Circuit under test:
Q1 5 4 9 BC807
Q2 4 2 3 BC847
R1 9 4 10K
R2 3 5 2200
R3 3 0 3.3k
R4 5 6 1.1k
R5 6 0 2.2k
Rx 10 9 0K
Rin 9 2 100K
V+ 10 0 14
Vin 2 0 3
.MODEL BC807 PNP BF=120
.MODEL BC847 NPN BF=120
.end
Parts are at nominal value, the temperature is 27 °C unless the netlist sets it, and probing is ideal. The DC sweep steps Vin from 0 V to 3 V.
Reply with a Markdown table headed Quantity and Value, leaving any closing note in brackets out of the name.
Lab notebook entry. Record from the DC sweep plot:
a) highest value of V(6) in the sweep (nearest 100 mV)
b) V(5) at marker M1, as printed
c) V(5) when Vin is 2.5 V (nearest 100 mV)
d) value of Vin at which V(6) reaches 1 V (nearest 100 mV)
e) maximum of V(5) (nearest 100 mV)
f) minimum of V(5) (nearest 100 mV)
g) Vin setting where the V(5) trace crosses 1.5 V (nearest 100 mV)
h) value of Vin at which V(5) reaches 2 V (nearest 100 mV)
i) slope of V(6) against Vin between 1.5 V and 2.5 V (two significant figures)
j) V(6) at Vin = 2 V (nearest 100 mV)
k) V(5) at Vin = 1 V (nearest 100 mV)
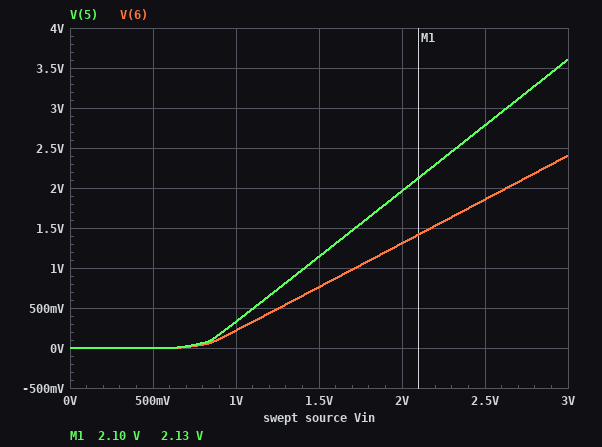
| Quantity | Value |
|---|---|
| highest value of V(6) in the sweep | 2.4 V |
| V(5) at marker M1, as printed | 2.13 V |
| V(5) when Vin is 2.5 V | 2.8 V |
| value of Vin at which V(6) reaches 1 V | 1.7 V |
| maximum of V(5) | 3.6 V |
| minimum of V(5) | 0 V |
| Vin setting where the V(5) trace crosses 1.5 V | 1.7 V |
| value of Vin at which V(5) reaches 2 V | 2.0 V |
| slope of V(6) against Vin between 1.5 V and 2.5 V | 1.1 V/V |
| V(6) at Vin = 2 V | 1.3 V |
| V(5) at Vin = 1 V | 300 mV |
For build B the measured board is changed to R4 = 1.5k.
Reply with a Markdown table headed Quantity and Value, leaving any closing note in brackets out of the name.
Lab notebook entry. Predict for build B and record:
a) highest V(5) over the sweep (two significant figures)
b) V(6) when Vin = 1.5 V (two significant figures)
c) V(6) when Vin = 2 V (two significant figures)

| Quantity | Value |
|---|---|
| highest V(5) over the sweep | 3.6 V |
| V(6) when Vin = 1.5 V | 680 mV |
| V(6) when Vin = 2 V | 1.2 V |
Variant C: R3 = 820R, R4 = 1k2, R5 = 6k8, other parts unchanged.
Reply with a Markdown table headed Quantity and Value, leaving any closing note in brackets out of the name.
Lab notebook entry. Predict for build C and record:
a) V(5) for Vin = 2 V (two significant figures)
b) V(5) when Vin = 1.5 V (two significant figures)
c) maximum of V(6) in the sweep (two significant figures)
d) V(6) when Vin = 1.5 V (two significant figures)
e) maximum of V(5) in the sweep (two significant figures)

| Quantity | Value |
|---|---|
| V(5) for Vin = 2 V | 4.5 V |
| V(5) when Vin = 1.5 V | 2.7 V |
| maximum of V(6) in the sweep | 6.9 V |
| V(6) when Vin = 1.5 V | 2.3 V |
| maximum of V(5) in the sweep | 8.2 V |
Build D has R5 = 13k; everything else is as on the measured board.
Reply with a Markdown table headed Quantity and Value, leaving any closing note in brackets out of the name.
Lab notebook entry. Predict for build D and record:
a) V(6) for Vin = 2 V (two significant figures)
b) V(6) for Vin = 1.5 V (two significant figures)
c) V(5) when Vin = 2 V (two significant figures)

| Quantity | Value |
|---|---|
| V(6) for Vin = 2 V | 1.8 V |
| V(6) for Vin = 1.5 V | 1.1 V |
| V(5) when Vin = 2 V | 2.0 V |
